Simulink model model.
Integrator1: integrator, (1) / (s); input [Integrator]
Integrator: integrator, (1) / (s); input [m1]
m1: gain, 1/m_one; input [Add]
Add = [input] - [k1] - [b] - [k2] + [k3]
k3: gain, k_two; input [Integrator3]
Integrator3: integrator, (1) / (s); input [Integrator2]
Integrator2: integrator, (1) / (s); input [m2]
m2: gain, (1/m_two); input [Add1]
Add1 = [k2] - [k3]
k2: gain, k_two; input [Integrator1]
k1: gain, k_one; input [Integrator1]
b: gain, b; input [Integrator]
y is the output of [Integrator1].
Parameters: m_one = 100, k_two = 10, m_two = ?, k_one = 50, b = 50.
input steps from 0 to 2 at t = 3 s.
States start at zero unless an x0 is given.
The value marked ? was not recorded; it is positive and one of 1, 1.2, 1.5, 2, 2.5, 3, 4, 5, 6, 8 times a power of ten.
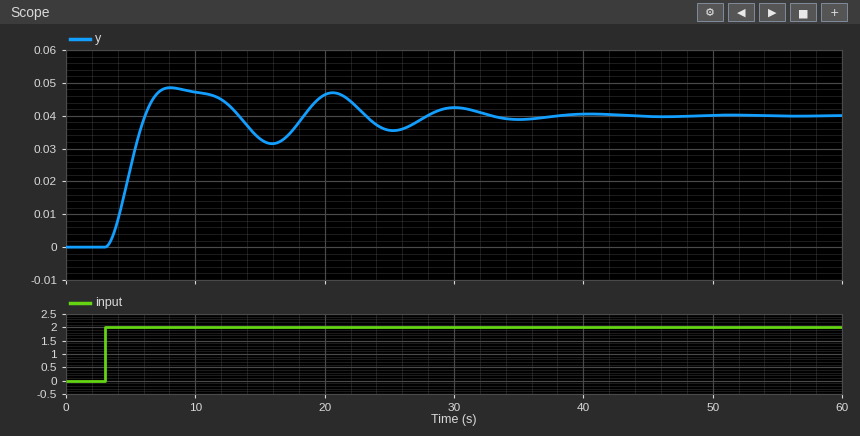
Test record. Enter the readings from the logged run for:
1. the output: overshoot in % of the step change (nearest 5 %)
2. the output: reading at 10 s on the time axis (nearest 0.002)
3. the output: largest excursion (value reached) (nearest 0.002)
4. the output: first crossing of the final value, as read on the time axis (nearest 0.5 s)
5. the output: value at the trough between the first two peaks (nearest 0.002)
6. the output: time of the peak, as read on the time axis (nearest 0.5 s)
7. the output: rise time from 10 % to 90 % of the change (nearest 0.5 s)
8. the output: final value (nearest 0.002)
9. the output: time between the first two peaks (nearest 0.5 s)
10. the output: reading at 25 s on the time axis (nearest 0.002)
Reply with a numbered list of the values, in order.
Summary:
1. 20 %
2. 0.048
3. 0.048
4. 6.0 s
5. 0.032
6. 8.0 s
7. 2.0 s
8. 0.040
9. 12.5 s
10. 0.036
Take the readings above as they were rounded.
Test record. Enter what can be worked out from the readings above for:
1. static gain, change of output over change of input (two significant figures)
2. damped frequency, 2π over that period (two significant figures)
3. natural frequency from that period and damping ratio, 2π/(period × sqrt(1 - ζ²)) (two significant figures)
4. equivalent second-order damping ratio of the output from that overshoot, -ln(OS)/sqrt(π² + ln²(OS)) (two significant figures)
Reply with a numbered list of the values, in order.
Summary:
1. 0.020
2. 0.50 rad/s
3. 0.57 rad/s
4. 0.46
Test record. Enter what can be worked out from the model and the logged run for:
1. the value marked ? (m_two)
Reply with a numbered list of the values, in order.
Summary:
1. 20
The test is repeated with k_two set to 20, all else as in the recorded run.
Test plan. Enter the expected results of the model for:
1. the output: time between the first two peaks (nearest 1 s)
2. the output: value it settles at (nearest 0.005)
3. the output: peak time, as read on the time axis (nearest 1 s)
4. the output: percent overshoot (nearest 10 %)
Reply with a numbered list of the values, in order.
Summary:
1. 8 s
2. 0.040
3. 9 s
4. 30 %
